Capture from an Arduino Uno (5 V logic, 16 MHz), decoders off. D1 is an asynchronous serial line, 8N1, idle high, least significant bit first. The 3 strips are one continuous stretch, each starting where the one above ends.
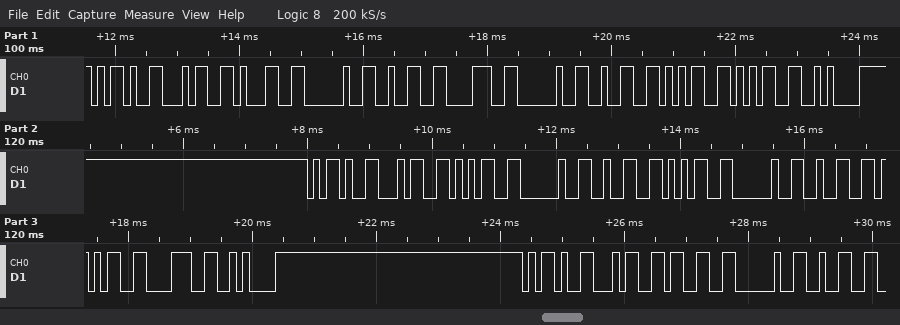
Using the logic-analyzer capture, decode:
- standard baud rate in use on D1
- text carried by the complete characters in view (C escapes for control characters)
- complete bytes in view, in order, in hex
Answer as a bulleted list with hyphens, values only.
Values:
- 9600 baud
- "-41 28 255\n-45 25 258\n-43 2"
- 2D 34 31 20 32 38 20 32 35 35 0A 2D 34 35 20 32 35 20 32 35 38 0A 2D 34 33 20 32
